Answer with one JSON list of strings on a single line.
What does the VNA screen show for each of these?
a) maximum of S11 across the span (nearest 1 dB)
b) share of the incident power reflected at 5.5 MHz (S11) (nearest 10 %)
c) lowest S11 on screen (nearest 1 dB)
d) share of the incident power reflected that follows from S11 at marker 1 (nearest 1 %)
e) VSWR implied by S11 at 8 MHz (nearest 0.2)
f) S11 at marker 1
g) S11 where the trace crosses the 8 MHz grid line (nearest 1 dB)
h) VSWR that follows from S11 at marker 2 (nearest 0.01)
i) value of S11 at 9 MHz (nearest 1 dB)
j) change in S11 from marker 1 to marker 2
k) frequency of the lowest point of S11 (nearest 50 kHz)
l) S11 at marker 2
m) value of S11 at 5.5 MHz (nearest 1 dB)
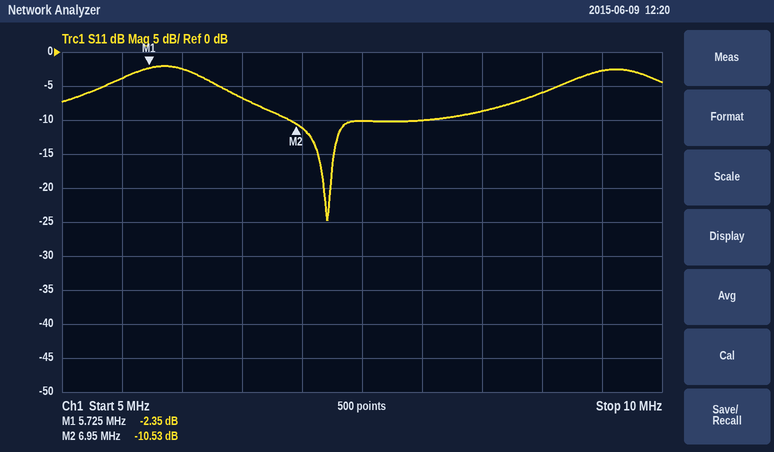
["-2 dB", "40 %", "-25 dB", "58 %", "2.0", "-2.35 dB", "-10 dB", "1.85", "-6 dB", "-8.18 dB", "7.20 MHz", "-10.53 dB", "-4 dB"]
